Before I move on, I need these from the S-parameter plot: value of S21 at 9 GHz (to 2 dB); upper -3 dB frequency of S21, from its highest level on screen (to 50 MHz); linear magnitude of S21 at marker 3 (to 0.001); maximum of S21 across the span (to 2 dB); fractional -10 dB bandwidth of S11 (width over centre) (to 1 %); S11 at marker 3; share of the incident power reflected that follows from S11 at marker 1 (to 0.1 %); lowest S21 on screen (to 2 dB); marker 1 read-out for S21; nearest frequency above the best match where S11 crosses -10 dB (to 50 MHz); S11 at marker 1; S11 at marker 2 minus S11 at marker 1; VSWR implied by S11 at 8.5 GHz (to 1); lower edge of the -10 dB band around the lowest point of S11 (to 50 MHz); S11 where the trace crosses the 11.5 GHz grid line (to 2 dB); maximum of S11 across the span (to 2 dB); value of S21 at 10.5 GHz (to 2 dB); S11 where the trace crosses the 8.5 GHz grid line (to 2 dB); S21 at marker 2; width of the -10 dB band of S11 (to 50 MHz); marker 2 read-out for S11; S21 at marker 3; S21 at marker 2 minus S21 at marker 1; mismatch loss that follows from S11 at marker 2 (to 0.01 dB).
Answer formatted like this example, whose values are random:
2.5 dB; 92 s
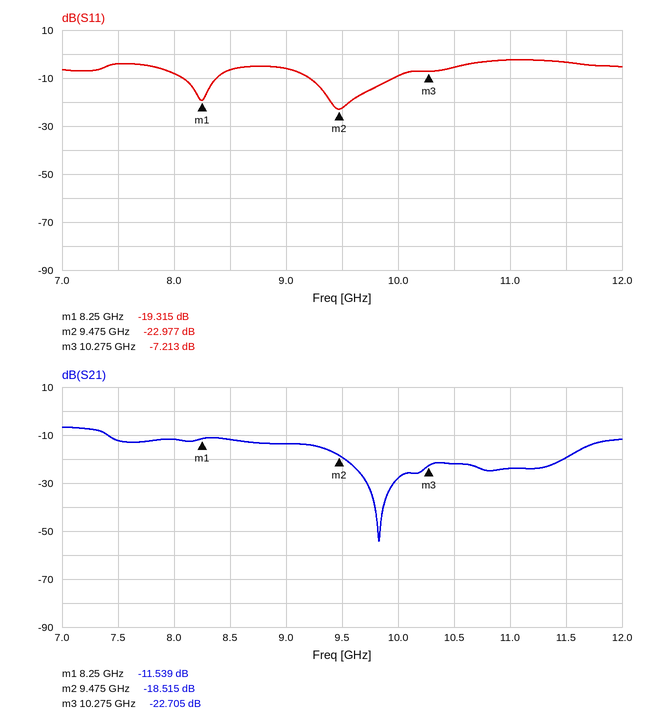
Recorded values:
-14 dB; 7.40 GHz; 0.073; -6 dB; 8 %; -7.213 dB; 1.2 %; -54 dB; -11.539 dB; 9.95 GHz; -19.315 dB; -3.662 dB; 3; 9.20 GHz; -4 dB; -2 dB; -22 dB; -6 dB; -18.515 dB; 750 MHz; -22.977 dB; -22.705 dB; -6.976 dB; 0.02 dB
